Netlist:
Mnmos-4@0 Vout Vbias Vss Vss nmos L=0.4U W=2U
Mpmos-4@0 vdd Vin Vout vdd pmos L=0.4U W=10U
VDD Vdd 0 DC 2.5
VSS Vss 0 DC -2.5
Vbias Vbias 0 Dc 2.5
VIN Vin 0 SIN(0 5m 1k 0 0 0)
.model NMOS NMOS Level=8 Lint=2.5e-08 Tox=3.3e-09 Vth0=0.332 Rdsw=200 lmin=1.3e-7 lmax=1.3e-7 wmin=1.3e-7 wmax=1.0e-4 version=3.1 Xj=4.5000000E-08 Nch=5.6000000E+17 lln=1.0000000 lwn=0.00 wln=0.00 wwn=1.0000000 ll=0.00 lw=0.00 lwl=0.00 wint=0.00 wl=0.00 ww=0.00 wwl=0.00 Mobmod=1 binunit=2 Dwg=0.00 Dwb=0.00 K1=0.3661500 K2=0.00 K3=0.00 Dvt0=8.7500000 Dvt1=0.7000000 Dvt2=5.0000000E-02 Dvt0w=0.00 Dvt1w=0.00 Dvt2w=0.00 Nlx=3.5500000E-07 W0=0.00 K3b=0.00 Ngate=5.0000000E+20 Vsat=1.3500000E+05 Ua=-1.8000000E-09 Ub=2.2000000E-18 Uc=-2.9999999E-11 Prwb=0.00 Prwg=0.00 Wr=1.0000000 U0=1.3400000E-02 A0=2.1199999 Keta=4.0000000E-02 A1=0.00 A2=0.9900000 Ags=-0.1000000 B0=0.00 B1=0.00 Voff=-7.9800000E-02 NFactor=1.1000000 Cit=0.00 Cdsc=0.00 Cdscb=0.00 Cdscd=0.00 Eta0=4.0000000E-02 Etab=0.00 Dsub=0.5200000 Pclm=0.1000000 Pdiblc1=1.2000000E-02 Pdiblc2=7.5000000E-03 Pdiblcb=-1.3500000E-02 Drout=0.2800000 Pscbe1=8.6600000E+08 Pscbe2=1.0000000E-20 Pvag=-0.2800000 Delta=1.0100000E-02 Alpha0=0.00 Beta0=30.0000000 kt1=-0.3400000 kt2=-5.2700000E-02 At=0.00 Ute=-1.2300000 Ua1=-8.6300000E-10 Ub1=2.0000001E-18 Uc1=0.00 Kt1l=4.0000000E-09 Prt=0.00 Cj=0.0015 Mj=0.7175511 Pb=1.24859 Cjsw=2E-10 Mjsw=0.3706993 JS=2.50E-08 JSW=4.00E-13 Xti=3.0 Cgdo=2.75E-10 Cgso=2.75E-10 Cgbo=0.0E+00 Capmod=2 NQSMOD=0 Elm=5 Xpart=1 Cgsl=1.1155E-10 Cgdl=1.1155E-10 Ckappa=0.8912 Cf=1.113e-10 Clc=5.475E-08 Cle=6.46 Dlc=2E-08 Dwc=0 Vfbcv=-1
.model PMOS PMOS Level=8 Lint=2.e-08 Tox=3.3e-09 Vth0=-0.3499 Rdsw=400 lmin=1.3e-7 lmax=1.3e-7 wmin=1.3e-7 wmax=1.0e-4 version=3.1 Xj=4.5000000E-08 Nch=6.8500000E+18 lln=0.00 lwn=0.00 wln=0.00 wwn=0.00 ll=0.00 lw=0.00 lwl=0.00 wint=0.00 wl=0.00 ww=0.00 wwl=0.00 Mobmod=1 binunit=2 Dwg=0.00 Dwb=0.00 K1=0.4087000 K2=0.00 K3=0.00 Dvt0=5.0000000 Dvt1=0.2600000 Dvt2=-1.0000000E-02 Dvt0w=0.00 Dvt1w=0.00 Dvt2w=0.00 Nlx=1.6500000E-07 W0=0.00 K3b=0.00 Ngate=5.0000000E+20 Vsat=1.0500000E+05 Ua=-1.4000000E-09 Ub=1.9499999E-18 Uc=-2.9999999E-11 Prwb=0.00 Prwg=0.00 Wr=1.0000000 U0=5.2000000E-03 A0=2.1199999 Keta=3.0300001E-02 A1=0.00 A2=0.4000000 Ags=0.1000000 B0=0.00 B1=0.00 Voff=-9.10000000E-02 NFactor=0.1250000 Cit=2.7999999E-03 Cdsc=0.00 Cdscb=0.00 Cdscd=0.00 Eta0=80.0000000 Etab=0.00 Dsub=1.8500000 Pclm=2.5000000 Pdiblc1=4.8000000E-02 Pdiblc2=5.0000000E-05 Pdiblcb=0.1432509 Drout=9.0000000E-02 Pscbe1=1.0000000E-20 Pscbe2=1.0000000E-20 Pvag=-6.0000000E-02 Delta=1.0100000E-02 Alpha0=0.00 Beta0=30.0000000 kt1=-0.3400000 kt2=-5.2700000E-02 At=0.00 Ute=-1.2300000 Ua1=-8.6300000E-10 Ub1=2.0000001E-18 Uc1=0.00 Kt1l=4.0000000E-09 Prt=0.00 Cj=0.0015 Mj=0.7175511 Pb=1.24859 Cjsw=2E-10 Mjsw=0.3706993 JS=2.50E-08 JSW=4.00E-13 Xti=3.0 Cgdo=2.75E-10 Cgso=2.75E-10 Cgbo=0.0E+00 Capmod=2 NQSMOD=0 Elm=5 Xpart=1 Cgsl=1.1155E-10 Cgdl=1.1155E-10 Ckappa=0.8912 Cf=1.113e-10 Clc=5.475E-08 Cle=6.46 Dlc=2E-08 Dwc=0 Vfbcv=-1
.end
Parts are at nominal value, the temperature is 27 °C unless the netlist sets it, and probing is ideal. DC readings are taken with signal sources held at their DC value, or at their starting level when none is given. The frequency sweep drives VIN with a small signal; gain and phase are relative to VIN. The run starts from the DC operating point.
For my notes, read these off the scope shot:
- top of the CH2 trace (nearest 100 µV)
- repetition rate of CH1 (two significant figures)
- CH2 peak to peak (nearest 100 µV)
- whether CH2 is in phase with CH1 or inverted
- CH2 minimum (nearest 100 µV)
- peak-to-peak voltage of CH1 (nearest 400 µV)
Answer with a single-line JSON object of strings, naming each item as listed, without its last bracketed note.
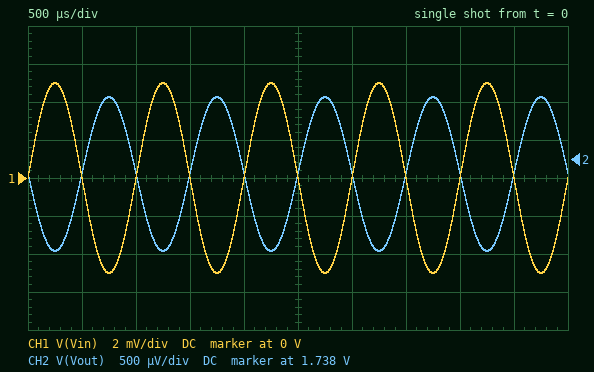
{"top of the CH2 trace": "1.7383 V", "repetition rate of CH1": "1.0 kHz", "CH2 peak to peak": "2.0 mV", "whether CH2 is in phase with CH1 or inverted": "inverted", "CH2 minimum": "1.7363 V", "peak-to-peak voltage of CH1": "10.0 mV"}
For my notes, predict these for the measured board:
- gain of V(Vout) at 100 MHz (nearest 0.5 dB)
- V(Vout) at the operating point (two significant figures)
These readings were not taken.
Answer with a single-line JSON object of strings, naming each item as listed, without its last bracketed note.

{"gain of V(Vout) at 100 MHz": "-14.0 dB", "V(Vout) at the operating point": "1.7 V"}
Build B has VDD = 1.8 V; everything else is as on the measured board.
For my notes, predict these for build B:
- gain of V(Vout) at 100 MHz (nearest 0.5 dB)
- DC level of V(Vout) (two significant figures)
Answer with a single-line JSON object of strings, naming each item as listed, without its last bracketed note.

{"gain of V(Vout) at 100 MHz": "11.5 dB", "DC level of V(Vout)": "-420 mV"}
